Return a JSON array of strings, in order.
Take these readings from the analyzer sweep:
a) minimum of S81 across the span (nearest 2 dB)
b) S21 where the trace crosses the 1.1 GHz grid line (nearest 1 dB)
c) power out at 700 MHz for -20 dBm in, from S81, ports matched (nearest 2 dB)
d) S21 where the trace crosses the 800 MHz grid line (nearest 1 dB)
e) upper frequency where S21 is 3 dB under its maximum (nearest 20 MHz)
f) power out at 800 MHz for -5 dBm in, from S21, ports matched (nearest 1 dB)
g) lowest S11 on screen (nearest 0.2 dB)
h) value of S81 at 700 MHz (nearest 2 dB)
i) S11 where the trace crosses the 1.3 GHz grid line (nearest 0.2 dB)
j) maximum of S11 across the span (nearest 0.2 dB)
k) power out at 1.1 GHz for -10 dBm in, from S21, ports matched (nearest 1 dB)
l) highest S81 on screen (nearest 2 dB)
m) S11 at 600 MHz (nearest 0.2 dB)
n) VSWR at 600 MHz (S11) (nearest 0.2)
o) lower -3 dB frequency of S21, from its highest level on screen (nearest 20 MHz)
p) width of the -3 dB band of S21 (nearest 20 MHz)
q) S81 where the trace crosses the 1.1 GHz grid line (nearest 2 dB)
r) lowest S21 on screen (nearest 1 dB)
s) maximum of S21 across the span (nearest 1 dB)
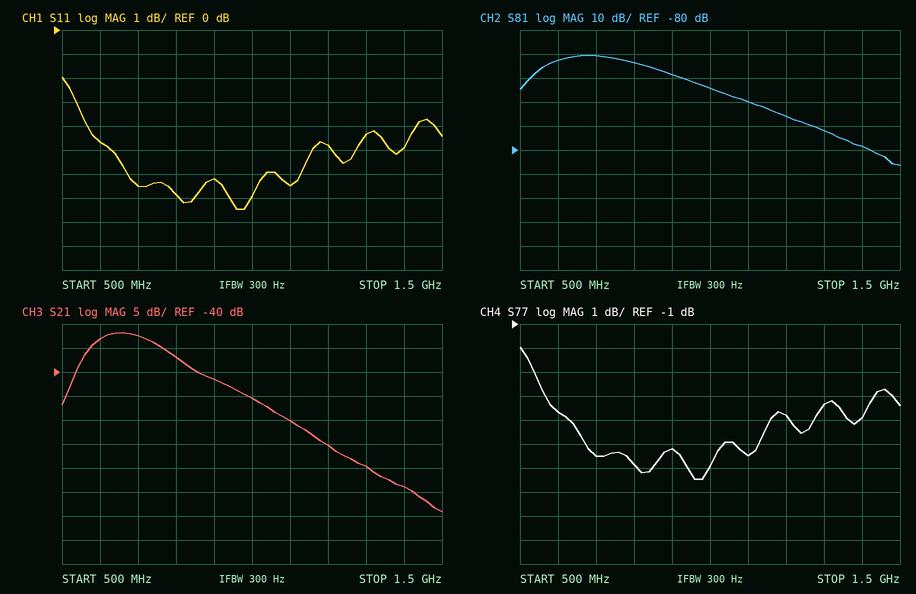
["-86 dB", "-50 dB", "-60 dBm", "-37 dB", "760 MHz", "-42 dBm", "-7.4 dB", "-40 dB", "-4.4 dB", "-2.0 dB", "-60 dBm", "-40 dB", "-4.6 dB", "3.8", "580 MHz", "180 MHz", "-60 dB", "-69 dB", "-32 dB"]
